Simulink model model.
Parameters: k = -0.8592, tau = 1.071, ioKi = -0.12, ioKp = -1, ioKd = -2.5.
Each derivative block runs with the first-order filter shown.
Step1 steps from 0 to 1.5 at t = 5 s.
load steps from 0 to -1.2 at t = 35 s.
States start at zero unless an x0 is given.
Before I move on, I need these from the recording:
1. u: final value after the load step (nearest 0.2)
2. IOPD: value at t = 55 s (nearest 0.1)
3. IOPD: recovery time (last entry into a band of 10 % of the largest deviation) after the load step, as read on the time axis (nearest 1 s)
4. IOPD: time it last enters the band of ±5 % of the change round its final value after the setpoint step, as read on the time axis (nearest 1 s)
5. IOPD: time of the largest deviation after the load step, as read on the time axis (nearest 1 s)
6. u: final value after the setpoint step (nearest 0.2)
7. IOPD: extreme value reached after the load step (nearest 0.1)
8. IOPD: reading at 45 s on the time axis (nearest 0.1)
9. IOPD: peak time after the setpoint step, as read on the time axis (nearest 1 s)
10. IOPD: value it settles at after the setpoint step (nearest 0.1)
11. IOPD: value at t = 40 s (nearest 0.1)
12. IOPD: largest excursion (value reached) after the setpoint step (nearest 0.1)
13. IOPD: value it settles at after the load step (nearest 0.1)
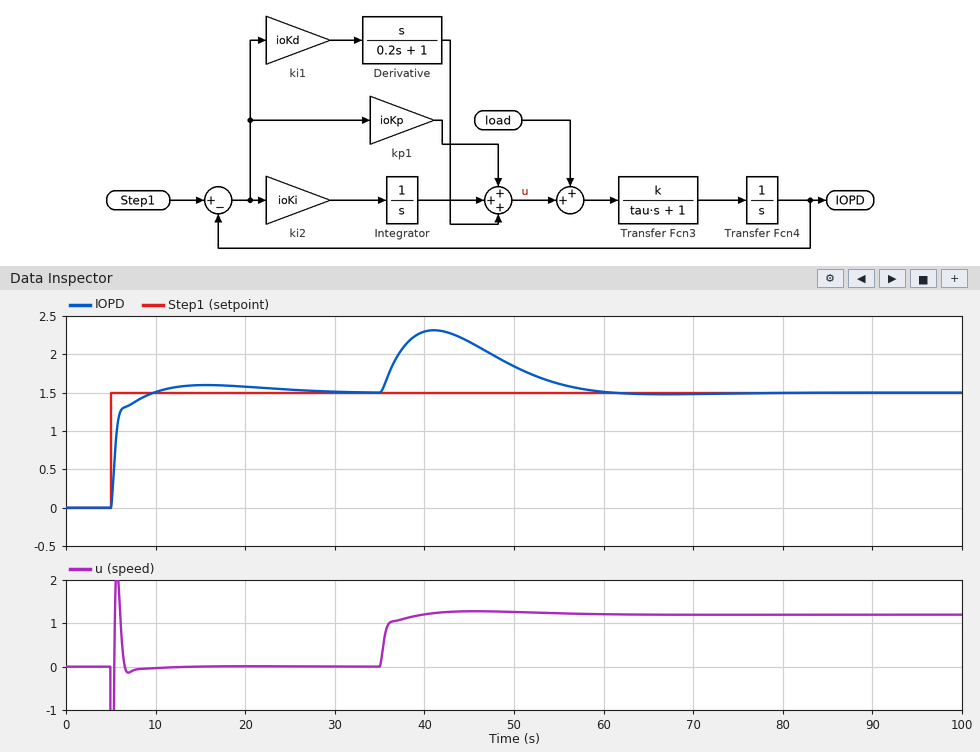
1.2
1.6
56 s
20 s
41 s
0.0
2.3
2.2
16 s
1.5
2.3
1.6
1.5
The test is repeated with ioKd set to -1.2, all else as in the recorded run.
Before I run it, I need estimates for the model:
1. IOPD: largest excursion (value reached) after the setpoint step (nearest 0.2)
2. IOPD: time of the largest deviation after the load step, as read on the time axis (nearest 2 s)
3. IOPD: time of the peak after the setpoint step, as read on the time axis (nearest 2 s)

1.6
40 s
12 s
